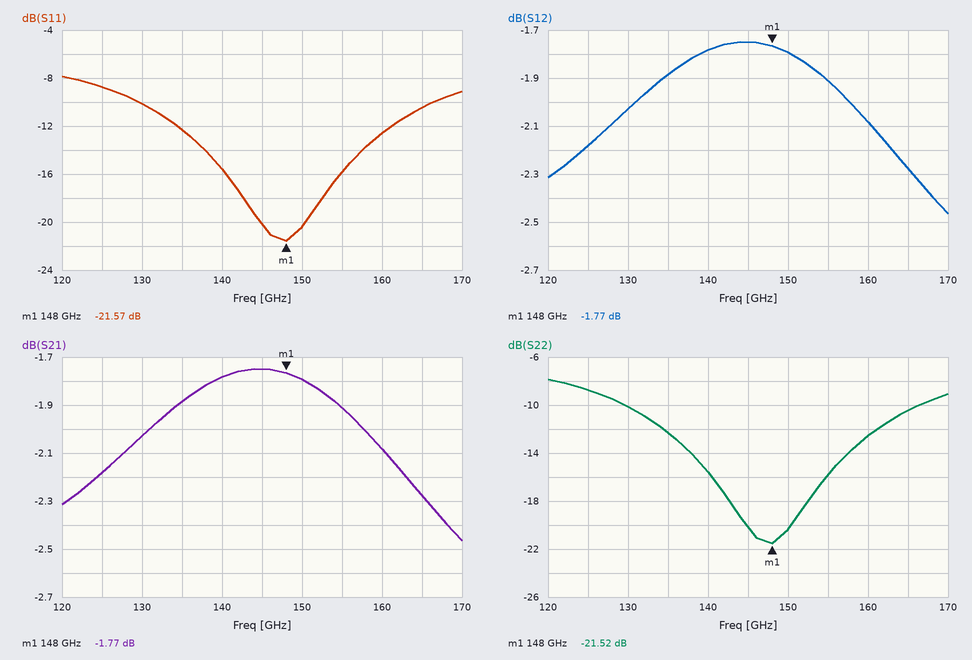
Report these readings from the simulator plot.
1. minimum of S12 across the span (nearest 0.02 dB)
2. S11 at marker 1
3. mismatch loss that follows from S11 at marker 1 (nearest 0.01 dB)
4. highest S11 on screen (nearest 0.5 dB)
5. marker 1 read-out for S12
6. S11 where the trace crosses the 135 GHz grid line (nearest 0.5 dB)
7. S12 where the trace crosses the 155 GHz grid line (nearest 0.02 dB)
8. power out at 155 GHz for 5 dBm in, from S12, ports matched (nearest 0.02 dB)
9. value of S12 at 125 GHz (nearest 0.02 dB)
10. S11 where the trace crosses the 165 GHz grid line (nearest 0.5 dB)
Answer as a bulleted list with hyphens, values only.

- -2.46 dB
- -21.57 dB
- 0.03 dB
- -8.0 dB
- -1.77 dB
- -12.5 dB
- -1.92 dB
- 3.08 dBm
- -2.18 dB
- -10.5 dB
